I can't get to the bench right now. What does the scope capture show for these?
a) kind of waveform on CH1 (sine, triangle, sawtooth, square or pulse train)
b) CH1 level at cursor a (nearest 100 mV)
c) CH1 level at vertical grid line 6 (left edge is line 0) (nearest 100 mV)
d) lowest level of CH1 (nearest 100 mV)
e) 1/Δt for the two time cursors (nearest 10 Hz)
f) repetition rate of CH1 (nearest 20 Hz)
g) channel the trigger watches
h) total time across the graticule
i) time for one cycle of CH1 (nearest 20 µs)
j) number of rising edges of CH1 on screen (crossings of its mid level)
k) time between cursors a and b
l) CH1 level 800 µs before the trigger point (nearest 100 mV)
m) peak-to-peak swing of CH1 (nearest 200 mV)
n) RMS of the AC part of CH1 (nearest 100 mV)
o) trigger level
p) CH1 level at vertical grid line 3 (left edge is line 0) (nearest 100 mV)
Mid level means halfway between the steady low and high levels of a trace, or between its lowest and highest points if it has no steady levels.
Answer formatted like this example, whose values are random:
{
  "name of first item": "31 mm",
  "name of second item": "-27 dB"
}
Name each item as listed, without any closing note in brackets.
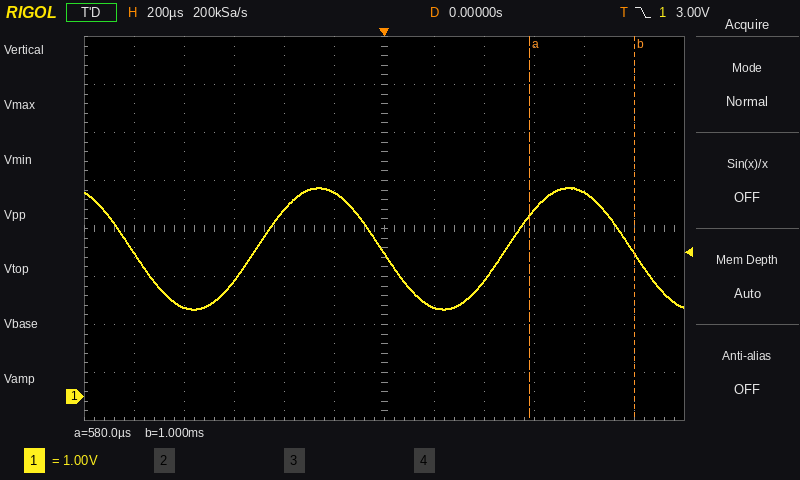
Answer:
{
  "kind of waveform on CH1": "sine",
  "CH1 level at cursor a": "3.8 V",
  "CH1 level at vertical grid line 6 (left edge is line 0)": "3.0 V",
  "lowest level of CH1": "1.8 V",
  "1/Δt for the two time cursors": "2.38 kHz",
  "repetition rate of CH1": "1.00 kHz",
  "channel the trigger watches": "CH1",
  "total time across the graticule": "2.4 ms",
  "time for one cycle of CH1": "1.00 ms",
  "number of rising edges of CH1 on screen": "2",
  "time between cursors a and b": "420 µs",
  "CH1 level 800 µs before the trigger point": "1.9 V",
  "peak-to-peak swing of CH1": "2.6 V",
  "RMS of the AC part of CH1": "900 mV",
  "trigger level": "3.00 V",
  "CH1 level at vertical grid line 3 (left edge is line 0)": "2.4 V"
}
